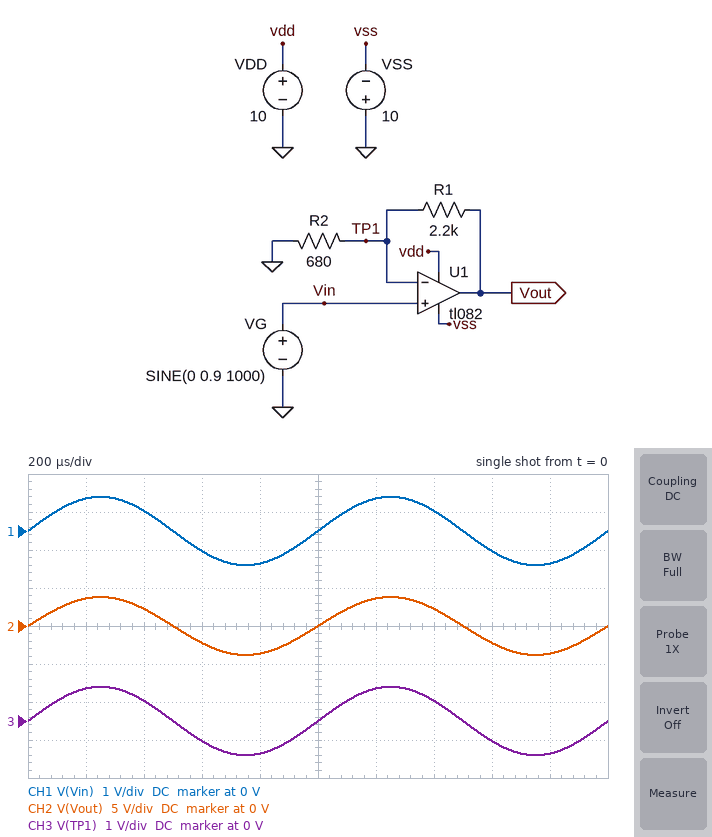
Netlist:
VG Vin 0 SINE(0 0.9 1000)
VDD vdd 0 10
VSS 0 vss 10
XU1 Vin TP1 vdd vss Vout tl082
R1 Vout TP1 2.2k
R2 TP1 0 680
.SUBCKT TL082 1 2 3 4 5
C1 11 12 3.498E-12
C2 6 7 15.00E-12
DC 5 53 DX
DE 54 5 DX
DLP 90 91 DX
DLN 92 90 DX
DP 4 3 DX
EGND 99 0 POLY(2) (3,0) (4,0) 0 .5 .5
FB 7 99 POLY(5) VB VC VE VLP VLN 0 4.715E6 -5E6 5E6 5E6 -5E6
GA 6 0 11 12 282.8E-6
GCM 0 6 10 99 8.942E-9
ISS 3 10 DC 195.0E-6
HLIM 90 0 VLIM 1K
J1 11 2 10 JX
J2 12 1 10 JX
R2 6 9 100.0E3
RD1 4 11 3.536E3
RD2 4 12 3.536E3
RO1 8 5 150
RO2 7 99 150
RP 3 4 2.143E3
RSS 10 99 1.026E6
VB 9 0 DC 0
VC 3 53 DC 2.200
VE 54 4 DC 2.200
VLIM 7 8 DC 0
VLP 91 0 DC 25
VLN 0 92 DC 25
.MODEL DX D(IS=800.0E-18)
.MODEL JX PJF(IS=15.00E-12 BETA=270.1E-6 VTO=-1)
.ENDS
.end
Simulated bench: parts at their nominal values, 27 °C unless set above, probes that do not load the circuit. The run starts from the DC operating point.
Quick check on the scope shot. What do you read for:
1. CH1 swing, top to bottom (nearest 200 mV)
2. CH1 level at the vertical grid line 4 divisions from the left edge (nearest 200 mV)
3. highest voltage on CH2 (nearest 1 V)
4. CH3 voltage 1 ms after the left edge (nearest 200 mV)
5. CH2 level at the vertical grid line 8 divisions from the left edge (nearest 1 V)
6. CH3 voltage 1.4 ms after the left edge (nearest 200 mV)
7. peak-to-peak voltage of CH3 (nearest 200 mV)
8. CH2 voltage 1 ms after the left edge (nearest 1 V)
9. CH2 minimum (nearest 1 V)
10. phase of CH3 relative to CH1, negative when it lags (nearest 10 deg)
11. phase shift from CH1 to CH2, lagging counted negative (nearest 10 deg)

1.8 V
-800 mV
4 V
0 V
-2 V
600 mV
1.8 V
0 V
-4 V
0 deg
0 deg
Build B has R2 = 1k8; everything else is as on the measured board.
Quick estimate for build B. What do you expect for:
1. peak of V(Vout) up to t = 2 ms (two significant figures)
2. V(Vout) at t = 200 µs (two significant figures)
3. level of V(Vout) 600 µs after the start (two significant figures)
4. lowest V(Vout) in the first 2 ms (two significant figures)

2.0 V
1.9 V
-1.2 V
-2.0 V
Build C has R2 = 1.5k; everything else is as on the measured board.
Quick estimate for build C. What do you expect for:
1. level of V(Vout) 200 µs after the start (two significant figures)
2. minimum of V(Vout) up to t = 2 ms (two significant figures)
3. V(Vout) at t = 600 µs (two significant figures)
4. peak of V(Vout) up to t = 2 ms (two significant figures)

2.1 V
-2.2 V
-1.3 V
2.2 V
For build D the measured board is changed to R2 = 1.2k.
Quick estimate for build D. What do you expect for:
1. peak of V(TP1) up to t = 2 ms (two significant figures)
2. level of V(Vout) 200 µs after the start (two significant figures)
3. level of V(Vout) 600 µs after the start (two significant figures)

900 mV
2.4 V
-1.5 V
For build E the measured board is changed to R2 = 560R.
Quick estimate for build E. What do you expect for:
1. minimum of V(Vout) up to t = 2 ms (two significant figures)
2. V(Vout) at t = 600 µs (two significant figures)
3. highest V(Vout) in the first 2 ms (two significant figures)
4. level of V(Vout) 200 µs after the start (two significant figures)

-4.4 V
-2.6 V
4.4 V
4.2 V
